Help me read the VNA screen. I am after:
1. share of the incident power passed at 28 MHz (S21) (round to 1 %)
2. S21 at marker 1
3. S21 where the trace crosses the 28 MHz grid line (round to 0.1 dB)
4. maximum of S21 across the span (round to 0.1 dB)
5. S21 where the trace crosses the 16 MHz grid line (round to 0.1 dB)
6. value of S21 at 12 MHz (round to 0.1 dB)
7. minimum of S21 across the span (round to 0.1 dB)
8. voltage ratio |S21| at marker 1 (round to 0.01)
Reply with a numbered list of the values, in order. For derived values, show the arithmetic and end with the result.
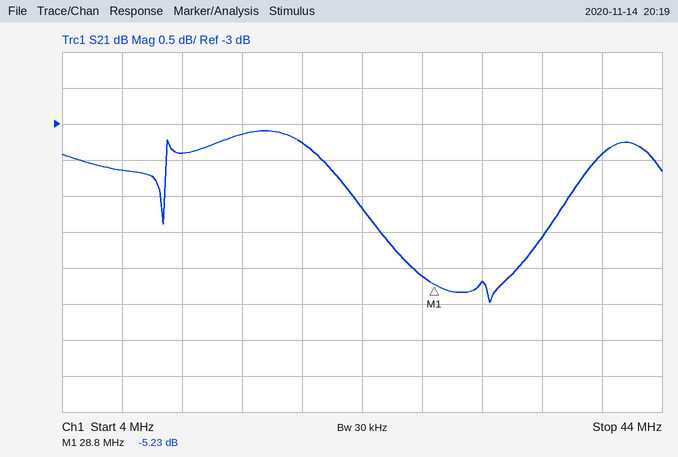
1. 10^(-5.1/10) ≈ 31 %
2. -5.23 dB
3. -5.1 dB
4. -3.1 dB
5. -3.1 dB
6. -3.4 dB
7. -5.5 dB
8. 10^(-5.23/20) ≈ 0.55
